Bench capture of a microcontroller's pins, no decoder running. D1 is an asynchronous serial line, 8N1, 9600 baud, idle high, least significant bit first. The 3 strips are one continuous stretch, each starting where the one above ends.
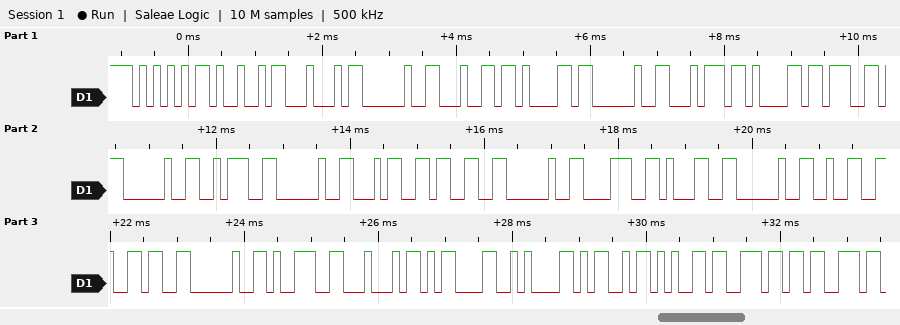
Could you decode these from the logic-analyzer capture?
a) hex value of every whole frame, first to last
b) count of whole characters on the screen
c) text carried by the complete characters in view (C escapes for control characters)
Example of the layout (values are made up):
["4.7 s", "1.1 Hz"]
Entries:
["55 49 44 20 64 61 20 74 61 67 20 3A 20 34 33 20 38 31 20 32 36 20 39 44 0D 0A 4D 65 6E 73", "30", "\"UID da tag : 43 81 26 9D\\r\\nMens\""]
